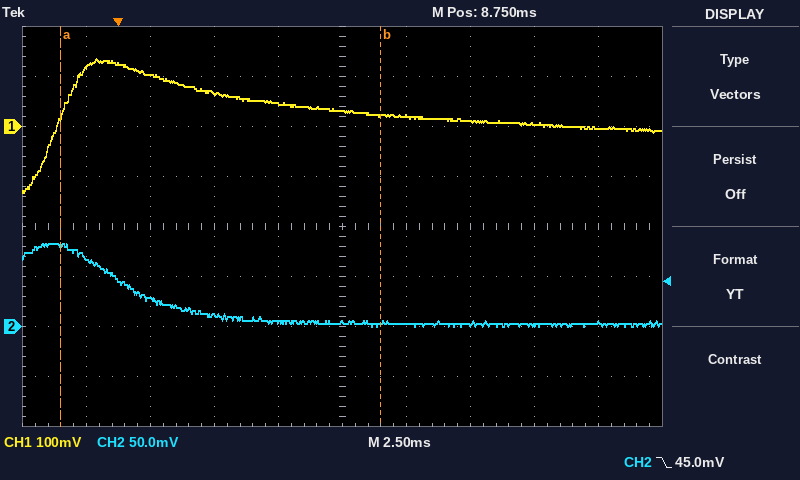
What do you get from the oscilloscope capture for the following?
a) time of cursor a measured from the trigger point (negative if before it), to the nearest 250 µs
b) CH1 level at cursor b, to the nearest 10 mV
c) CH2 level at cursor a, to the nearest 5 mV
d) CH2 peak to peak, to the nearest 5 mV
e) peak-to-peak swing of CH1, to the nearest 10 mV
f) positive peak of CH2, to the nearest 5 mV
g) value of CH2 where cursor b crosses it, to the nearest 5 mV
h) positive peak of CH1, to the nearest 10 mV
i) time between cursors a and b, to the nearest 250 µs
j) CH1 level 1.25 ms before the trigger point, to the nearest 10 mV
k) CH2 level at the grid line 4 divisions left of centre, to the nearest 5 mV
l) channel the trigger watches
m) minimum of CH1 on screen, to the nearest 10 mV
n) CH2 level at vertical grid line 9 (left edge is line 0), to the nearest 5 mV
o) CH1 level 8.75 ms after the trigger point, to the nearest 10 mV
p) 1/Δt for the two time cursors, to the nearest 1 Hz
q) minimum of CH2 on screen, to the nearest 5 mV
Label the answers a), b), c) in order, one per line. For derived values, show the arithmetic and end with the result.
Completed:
a) -2.25 ms
b) 20 mV
c) 80 mV
d) 85 mV − (0 mV) = 85 mV
e) 140 mV − (-130 mV) = 270 mV
f) 85 mV
g) 5 mV
h) 140 mV
i) 12.50 ms
j) 120 mV
k) 70 mV
l) CH2
m) -130 mV
n) 5 mV
o) 30 mV
p) 1 / 12.50 ms ≈ 80 Hz
q) 0 mV
